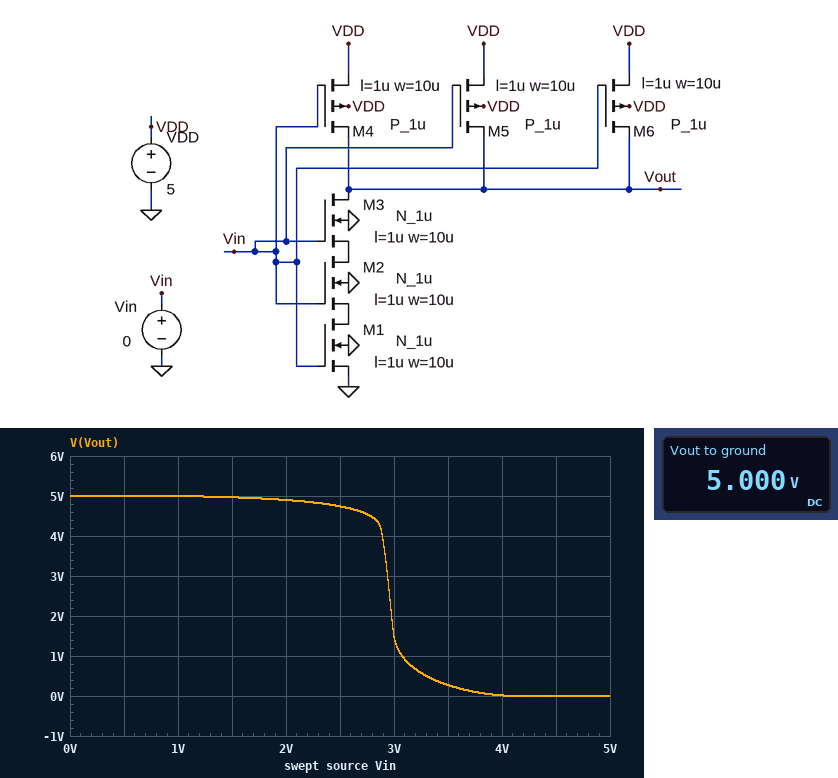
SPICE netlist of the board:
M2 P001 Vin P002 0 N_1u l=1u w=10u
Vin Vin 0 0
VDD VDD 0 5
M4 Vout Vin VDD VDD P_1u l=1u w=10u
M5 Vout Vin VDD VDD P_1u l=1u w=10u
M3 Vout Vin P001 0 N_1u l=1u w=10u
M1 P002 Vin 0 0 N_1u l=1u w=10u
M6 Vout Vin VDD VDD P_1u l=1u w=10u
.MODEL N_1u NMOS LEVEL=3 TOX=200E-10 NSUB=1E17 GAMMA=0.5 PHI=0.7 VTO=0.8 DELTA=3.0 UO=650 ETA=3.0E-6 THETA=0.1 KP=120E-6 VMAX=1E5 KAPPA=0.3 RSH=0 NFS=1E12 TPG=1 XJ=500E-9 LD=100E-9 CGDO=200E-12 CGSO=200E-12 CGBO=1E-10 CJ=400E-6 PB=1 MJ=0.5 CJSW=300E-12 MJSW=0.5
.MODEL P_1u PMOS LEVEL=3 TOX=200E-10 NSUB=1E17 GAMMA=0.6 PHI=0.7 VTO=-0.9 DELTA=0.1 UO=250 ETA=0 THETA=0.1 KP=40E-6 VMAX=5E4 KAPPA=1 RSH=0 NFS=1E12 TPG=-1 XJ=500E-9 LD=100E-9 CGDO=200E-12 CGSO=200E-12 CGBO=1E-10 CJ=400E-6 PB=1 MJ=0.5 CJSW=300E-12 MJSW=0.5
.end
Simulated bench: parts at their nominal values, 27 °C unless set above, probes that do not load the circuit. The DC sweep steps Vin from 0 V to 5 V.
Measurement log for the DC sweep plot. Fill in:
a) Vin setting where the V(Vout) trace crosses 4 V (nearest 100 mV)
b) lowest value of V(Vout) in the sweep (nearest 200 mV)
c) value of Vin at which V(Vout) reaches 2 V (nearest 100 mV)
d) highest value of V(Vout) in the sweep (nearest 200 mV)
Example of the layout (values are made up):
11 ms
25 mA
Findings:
2.9 V
0 V
3.0 V
5.0 V
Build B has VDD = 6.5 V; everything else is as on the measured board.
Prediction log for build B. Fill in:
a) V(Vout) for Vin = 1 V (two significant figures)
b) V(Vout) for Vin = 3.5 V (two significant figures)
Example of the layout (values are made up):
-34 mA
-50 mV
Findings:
6.5 V
6.0 V
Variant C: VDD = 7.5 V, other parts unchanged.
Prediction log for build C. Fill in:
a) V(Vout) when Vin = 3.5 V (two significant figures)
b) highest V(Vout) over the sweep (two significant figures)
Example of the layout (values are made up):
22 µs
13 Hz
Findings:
7.2 V
7.5 V
